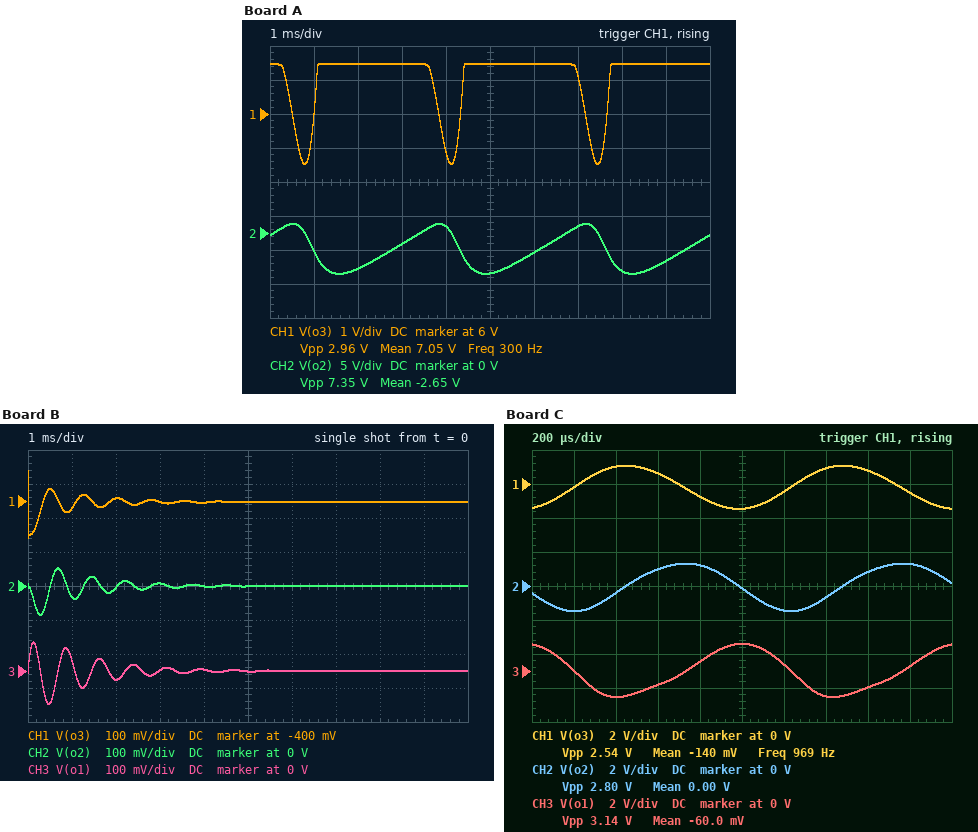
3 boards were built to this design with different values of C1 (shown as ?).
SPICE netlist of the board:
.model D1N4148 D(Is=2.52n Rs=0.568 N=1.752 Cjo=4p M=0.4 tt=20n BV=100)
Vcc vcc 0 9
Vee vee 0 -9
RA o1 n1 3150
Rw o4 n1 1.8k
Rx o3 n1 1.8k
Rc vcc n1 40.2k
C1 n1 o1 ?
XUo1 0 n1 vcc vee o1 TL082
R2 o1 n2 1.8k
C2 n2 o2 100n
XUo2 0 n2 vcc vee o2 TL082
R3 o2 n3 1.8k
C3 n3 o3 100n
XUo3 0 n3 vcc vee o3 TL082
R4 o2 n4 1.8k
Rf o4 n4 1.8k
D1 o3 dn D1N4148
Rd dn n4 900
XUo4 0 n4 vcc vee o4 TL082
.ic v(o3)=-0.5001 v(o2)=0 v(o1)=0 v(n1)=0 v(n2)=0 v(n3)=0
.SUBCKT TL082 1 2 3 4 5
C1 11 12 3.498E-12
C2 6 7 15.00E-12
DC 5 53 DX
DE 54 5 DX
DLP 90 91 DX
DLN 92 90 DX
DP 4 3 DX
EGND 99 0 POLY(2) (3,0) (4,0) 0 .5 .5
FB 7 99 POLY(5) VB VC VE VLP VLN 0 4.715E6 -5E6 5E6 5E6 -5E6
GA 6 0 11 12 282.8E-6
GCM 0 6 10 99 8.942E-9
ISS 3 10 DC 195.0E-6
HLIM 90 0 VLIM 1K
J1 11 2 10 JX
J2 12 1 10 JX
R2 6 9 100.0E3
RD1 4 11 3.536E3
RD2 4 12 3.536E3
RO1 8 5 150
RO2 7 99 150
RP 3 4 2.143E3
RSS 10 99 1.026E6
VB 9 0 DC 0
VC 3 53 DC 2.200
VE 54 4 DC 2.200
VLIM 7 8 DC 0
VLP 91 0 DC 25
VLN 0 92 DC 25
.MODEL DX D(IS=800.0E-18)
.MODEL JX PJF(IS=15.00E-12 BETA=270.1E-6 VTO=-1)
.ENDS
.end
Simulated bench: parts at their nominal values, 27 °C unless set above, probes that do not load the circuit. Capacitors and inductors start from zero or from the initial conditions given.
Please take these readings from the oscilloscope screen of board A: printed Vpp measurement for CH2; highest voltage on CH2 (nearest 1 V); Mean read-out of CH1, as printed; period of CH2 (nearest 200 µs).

7.35 V
1 V
7.05 V
3.4 ms
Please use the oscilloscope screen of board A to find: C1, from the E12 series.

120 nF
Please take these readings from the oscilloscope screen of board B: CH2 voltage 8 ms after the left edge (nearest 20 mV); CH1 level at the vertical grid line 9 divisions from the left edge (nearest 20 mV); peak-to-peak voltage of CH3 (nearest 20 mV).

0 V
-400 mV
180 mV
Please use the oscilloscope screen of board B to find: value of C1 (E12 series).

39 nF
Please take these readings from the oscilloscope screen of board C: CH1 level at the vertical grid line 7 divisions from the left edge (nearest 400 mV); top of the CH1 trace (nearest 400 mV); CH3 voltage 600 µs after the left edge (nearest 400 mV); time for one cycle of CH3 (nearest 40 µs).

800 mV
1.2 V
-800 mV
1.04 ms
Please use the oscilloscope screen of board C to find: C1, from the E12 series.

82 nF
